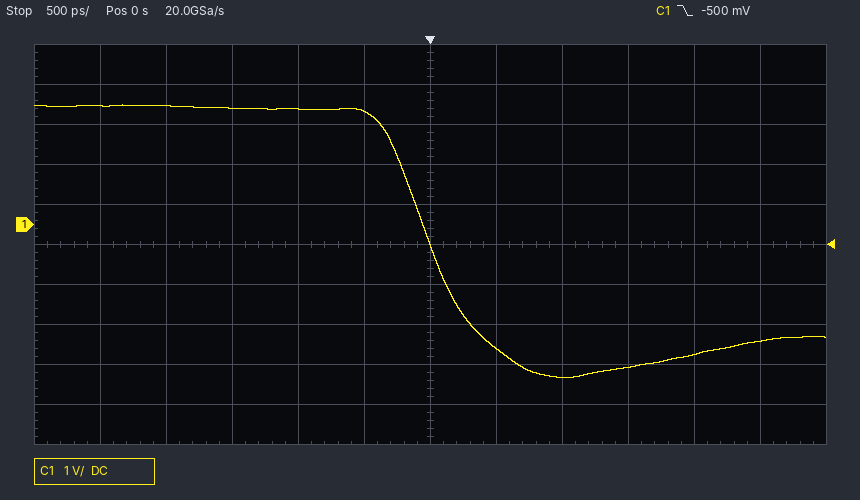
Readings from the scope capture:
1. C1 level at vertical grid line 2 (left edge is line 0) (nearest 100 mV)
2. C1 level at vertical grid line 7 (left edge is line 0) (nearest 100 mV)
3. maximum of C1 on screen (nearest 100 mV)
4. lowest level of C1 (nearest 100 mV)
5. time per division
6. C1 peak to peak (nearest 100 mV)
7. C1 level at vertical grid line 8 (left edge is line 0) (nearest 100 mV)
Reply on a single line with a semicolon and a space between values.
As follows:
3.0 V; -3.1 V; 3.0 V; -3.8 V; 500 ps; 6.8 V; -3.8 V
